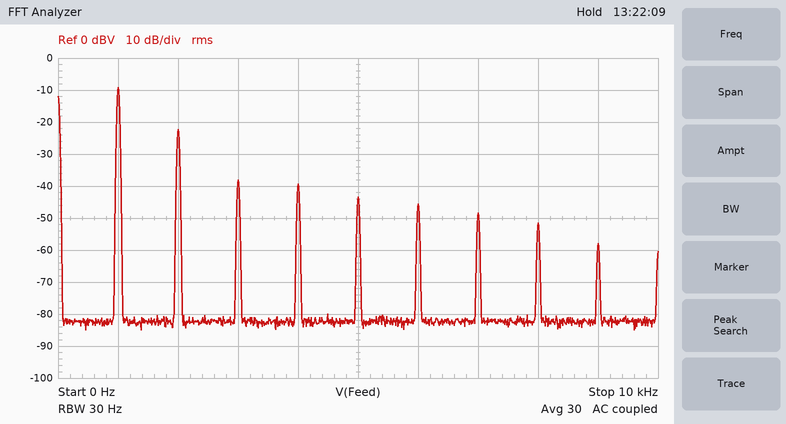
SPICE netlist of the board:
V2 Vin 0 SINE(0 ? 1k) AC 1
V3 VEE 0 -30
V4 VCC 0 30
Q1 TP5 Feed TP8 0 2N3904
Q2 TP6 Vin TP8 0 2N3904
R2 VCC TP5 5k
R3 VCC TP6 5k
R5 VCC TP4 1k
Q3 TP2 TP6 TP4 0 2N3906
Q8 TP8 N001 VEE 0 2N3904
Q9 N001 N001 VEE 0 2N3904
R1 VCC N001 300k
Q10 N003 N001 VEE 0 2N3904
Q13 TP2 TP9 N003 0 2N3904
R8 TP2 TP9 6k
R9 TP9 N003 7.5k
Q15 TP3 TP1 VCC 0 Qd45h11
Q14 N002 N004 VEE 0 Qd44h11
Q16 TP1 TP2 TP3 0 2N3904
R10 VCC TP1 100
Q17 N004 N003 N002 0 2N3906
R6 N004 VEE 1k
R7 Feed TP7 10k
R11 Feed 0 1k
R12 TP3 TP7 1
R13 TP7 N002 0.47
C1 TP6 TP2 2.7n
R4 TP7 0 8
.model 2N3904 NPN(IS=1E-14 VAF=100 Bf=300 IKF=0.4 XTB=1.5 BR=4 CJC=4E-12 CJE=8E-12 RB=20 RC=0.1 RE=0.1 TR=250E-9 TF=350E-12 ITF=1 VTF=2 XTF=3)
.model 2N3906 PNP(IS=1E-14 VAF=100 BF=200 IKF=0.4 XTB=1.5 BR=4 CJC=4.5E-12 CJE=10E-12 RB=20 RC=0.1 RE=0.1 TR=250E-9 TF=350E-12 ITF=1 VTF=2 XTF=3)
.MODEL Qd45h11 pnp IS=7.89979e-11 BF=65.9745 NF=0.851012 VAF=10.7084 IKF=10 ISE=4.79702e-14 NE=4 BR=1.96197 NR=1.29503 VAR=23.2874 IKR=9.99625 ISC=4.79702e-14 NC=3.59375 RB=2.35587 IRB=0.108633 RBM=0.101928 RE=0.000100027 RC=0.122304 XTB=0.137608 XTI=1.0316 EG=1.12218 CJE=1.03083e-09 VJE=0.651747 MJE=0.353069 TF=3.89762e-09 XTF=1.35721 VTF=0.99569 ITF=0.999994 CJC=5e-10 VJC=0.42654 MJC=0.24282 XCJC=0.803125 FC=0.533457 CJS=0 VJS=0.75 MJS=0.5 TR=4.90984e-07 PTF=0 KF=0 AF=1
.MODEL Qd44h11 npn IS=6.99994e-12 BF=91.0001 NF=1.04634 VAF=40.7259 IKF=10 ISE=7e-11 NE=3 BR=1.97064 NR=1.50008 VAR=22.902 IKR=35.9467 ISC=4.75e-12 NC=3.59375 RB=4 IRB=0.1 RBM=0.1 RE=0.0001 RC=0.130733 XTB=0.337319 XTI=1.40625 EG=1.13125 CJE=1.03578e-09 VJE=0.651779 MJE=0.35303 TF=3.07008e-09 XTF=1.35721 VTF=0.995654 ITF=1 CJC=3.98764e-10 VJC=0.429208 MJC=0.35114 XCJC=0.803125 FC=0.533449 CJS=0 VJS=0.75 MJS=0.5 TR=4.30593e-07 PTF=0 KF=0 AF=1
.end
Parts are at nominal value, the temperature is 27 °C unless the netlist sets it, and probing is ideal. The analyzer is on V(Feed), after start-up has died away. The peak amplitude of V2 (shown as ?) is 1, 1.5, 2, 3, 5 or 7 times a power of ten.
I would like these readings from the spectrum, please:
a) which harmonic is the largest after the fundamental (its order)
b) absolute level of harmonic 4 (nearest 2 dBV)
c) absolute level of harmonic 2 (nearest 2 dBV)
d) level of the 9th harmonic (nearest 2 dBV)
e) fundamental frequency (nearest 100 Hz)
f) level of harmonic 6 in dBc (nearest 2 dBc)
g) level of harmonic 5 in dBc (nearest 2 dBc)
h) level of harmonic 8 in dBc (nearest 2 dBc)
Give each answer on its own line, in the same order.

2
-40 dBV
-22 dBV
-58 dBV
1.0 kHz
-36 dBc
-34 dBc
-42 dBc
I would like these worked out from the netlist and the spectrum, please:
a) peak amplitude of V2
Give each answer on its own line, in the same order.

700 mV
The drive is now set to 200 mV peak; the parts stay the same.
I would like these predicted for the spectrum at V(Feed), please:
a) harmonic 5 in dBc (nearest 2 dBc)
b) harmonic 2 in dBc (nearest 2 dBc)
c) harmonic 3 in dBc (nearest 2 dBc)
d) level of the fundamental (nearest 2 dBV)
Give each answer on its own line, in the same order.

-46 dBc
-34 dBc
-38 dBc
-18 dBV
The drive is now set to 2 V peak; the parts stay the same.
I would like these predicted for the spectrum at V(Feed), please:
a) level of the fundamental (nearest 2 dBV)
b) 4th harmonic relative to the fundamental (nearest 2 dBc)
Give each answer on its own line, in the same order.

-8 dBV
-24 dBc
